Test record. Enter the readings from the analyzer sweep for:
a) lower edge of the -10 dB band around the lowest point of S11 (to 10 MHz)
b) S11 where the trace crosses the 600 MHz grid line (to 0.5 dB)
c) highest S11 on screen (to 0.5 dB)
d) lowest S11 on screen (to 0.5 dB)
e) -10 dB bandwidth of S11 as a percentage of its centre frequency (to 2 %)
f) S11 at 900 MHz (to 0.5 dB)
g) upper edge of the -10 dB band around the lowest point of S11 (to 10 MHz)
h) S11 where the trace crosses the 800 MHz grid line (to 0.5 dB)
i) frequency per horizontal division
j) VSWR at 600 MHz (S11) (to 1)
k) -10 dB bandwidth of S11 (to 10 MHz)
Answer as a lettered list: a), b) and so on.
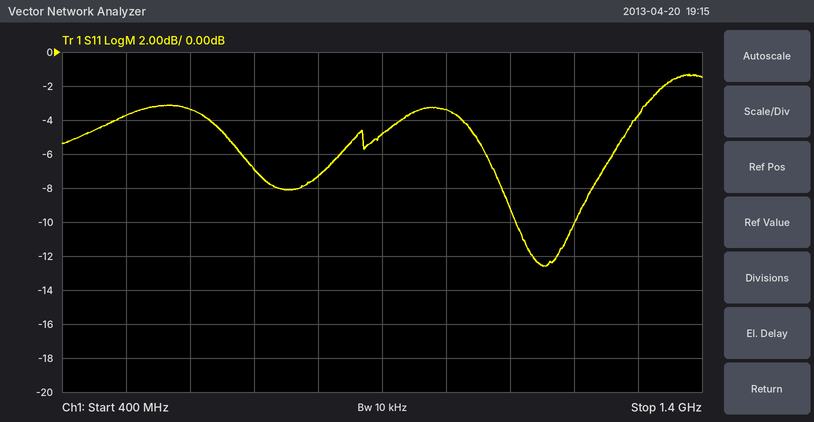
a) 1.11 GHz
b) -3.5 dB
c) -1.5 dB
d) -12.5 dB
e) 8 %
f) -5.0 dB
g) 1.20 GHz
h) -7.5 dB
i) 100 MHz
j) 5
k) 90 MHz
